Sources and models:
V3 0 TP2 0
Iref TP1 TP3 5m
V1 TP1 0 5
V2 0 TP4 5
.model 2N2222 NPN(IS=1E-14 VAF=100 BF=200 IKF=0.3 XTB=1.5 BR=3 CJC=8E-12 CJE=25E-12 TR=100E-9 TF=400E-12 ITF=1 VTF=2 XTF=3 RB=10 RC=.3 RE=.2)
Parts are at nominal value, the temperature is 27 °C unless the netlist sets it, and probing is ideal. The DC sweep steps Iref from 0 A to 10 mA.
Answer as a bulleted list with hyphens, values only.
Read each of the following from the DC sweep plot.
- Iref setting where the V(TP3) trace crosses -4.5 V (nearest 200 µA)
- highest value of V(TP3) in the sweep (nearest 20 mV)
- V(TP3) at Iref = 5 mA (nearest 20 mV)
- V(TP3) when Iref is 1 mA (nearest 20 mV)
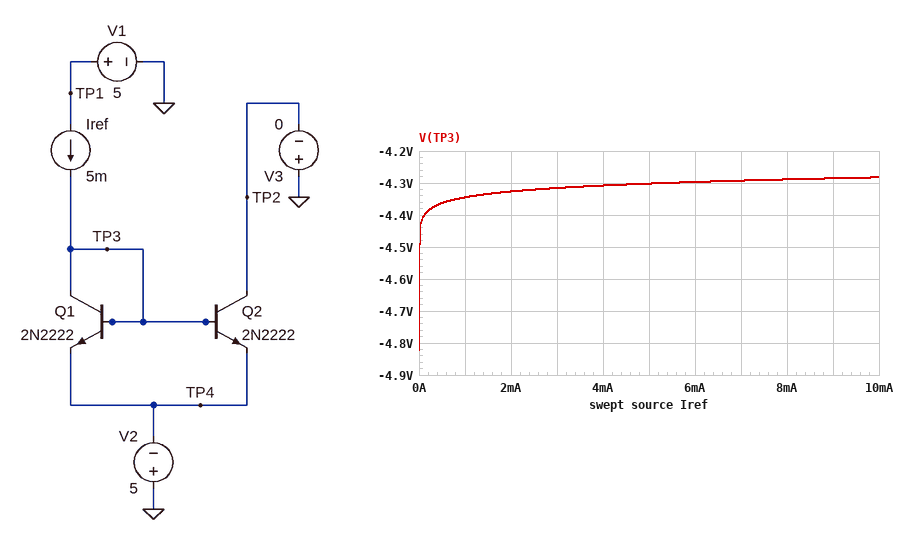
- 0 A
- -4.28 V
- -4.30 V
- -4.34 V
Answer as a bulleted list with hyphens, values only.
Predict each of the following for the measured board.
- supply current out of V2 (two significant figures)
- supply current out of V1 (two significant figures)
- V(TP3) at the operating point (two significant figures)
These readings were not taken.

- 10 mA
- 5.0 mA
- -4.3 V
